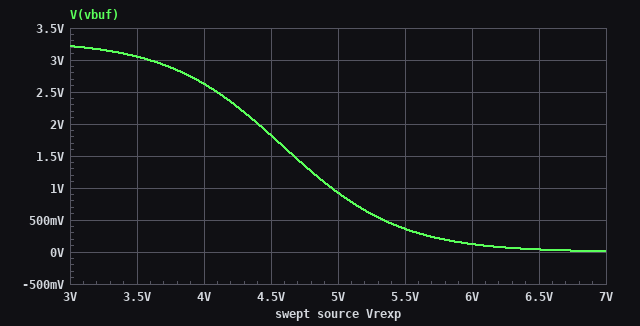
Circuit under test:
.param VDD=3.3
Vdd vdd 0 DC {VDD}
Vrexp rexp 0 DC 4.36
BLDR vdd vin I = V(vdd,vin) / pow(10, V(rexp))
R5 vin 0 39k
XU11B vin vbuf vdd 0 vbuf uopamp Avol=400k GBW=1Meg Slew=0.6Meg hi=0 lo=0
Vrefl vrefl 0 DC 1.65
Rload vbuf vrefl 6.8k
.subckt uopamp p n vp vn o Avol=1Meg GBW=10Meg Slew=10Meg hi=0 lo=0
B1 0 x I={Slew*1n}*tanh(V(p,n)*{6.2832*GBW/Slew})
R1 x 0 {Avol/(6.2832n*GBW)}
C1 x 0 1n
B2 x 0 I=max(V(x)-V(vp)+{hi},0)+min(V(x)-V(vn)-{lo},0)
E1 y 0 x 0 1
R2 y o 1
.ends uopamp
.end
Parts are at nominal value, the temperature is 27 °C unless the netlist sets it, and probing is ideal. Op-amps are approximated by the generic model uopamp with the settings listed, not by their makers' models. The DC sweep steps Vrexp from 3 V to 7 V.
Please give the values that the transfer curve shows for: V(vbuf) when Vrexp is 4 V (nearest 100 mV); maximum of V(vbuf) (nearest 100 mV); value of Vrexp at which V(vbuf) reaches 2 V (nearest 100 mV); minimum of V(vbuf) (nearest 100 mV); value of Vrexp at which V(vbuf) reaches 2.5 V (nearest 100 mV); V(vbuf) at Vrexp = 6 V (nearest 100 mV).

2.6 V
3.2 V
4.4 V
0 V
4.1 V
100 mV
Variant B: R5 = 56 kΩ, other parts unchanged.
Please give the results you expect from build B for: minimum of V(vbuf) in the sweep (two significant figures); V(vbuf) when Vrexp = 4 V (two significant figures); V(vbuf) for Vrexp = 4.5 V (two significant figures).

18 mV
2.8 V
2.1 V
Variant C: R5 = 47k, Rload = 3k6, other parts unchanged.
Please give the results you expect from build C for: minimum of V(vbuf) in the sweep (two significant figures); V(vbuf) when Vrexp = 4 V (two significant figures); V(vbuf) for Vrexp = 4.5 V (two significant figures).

15 mV
2.7 V
2.0 V
